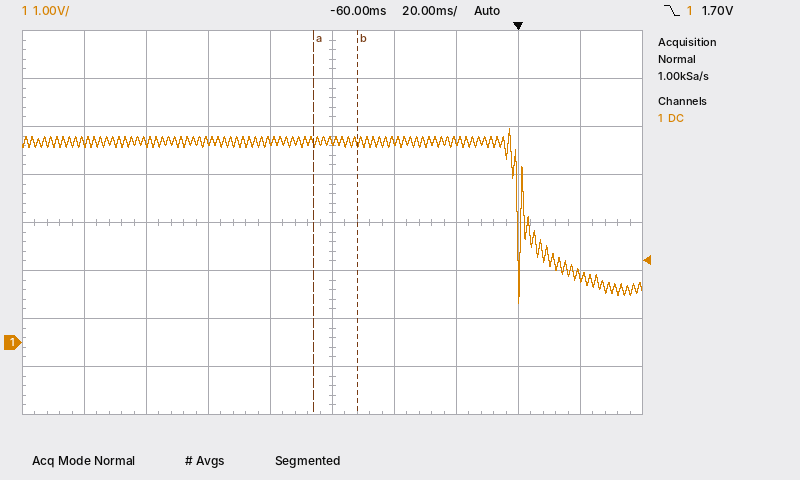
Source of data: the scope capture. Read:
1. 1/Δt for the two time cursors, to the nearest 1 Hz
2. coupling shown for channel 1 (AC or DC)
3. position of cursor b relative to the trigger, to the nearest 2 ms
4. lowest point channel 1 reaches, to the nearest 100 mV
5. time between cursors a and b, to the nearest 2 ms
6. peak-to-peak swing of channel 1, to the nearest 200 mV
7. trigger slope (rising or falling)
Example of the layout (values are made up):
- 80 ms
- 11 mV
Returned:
- 71 Hz
- DC
- -52 ms
- 800 mV
- 14 ms
- 3.6 V
- falling
